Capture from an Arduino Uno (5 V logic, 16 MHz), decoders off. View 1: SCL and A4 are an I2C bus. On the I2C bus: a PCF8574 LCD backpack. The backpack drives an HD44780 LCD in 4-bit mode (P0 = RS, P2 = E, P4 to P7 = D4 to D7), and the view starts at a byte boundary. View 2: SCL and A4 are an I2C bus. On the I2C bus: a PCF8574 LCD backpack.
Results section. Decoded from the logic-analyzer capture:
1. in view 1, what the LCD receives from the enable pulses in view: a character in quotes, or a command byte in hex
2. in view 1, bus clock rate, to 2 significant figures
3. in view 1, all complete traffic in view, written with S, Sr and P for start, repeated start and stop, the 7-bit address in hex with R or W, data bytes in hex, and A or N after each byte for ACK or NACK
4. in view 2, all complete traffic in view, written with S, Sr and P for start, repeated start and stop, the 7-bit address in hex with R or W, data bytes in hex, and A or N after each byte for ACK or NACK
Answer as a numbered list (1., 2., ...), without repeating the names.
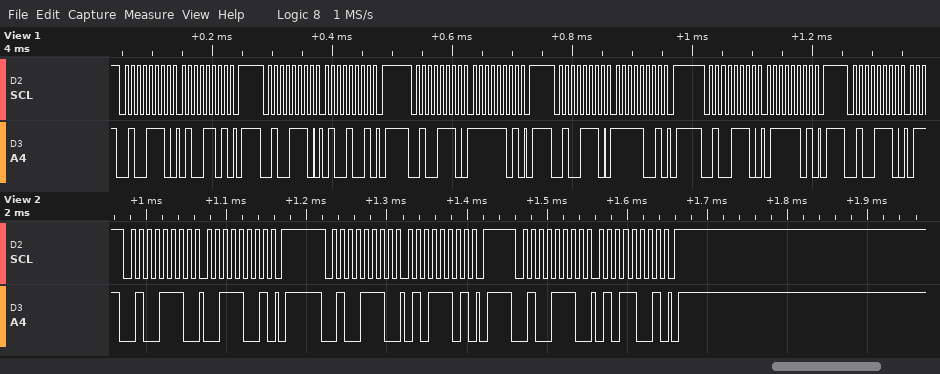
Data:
1. 'O'
2. 100 kHz
3. S 27W A 4D A P S 27W A 49 A P S 27W A FD A P S 27W A F9 A P S 27W A 7D A P S 27W A
4. S 27W A 39 A P S 27W A 5D A P S 27W A 59 A P
